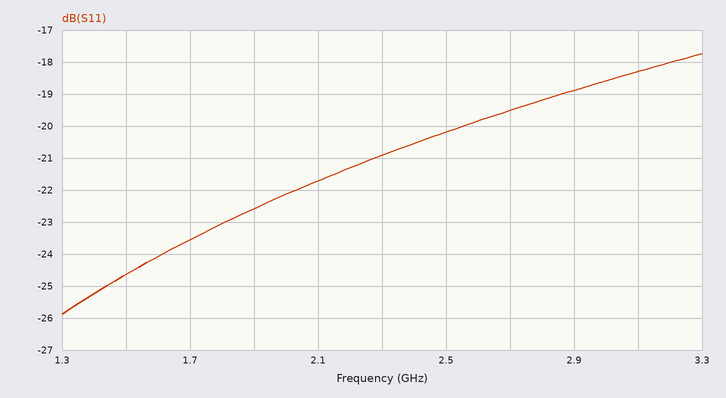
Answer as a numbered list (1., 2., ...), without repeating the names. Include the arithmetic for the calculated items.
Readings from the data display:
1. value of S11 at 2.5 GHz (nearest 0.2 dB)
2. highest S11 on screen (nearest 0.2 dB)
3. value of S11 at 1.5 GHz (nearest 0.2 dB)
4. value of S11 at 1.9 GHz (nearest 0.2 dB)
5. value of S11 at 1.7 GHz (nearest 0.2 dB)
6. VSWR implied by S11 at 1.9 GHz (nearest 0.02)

1. -20.2 dB
2. -17.8 dB
3. -24.6 dB
4. -22.6 dB
5. -23.6 dB
6. |Γ| = 10^(-22.6/20) = 0.0741; VSWR = (1 + 0.0741)/(1 − 0.0741) ≈ 1.16
